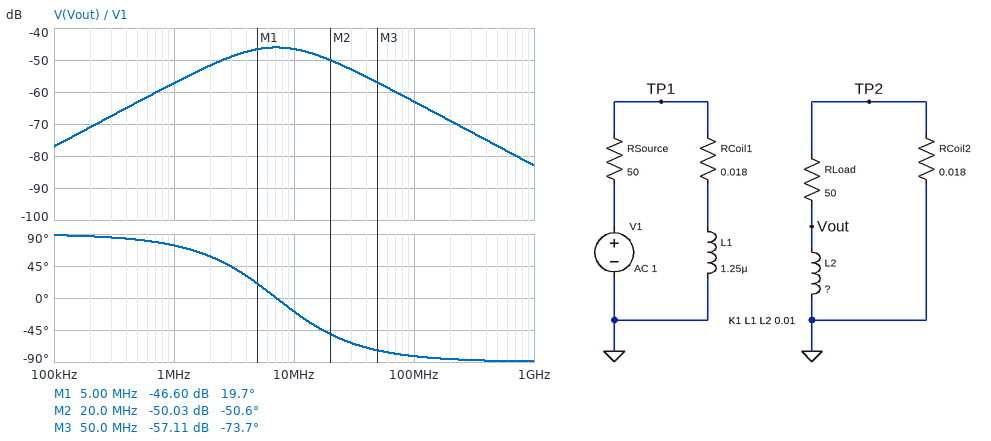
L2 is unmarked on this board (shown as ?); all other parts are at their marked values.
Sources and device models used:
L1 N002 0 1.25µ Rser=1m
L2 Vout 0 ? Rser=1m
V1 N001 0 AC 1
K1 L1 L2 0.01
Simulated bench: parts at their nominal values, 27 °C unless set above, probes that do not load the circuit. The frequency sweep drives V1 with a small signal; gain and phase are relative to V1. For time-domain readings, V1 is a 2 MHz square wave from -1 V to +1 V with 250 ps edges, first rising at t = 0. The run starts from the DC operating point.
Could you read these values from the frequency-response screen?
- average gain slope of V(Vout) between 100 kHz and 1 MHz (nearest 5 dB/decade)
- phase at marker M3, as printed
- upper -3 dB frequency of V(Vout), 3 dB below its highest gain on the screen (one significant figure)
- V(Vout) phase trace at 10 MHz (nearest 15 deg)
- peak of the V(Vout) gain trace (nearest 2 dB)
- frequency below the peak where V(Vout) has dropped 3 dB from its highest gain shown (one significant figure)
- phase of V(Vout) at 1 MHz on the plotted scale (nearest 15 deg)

20 dB/decade
-73.7 deg
20 MHz
-15 deg
-46 dB
3 MHz
75 deg
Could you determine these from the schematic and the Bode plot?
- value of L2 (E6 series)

1 µH
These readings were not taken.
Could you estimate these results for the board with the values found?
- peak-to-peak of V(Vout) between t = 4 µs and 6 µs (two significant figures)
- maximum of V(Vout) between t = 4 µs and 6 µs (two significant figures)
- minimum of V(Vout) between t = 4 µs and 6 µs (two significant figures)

15 mV
7.3 mV
-7.3 mV
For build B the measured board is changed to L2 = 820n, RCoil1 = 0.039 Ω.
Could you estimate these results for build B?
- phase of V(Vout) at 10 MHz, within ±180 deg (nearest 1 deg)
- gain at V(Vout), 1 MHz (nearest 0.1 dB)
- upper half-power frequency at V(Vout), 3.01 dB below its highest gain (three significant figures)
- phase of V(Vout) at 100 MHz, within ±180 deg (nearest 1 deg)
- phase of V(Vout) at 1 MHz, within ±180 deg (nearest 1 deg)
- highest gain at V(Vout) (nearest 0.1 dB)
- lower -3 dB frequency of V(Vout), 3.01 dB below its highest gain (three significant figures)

-13 deg
-58.1 dB
19.3 MHz
-81 deg
75 deg
-46.2 dB
3.21 MHz
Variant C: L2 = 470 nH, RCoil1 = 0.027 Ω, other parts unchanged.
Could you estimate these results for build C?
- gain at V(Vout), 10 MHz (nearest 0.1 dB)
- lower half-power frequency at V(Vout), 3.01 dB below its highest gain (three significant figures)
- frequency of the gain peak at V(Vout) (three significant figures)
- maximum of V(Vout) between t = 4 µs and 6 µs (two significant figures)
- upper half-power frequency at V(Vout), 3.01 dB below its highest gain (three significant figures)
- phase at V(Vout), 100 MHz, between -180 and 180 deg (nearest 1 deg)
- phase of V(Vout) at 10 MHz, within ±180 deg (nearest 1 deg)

-47.0 dB
3.96 MHz
10.4 MHz
6.8 mV
27.3 MHz
-77 deg
2 deg
